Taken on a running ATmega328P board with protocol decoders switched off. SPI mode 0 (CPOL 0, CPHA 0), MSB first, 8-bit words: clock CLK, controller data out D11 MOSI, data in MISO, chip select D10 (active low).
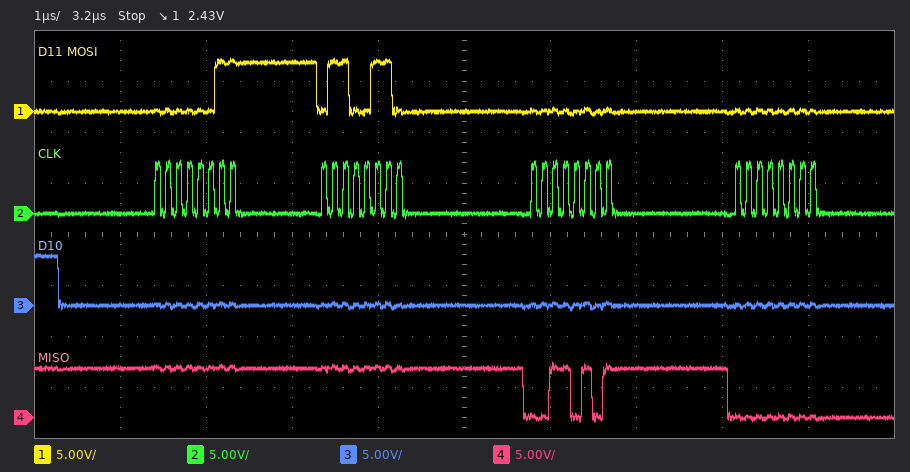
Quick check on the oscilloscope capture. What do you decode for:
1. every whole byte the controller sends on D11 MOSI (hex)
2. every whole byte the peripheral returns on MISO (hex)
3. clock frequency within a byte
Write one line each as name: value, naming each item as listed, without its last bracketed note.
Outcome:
every whole byte the controller sends on D11 MOSI: 03 66 00 00
every whole byte the peripheral returns on MISO: FF FF 35 00
clock frequency within a byte: 8 MHz
